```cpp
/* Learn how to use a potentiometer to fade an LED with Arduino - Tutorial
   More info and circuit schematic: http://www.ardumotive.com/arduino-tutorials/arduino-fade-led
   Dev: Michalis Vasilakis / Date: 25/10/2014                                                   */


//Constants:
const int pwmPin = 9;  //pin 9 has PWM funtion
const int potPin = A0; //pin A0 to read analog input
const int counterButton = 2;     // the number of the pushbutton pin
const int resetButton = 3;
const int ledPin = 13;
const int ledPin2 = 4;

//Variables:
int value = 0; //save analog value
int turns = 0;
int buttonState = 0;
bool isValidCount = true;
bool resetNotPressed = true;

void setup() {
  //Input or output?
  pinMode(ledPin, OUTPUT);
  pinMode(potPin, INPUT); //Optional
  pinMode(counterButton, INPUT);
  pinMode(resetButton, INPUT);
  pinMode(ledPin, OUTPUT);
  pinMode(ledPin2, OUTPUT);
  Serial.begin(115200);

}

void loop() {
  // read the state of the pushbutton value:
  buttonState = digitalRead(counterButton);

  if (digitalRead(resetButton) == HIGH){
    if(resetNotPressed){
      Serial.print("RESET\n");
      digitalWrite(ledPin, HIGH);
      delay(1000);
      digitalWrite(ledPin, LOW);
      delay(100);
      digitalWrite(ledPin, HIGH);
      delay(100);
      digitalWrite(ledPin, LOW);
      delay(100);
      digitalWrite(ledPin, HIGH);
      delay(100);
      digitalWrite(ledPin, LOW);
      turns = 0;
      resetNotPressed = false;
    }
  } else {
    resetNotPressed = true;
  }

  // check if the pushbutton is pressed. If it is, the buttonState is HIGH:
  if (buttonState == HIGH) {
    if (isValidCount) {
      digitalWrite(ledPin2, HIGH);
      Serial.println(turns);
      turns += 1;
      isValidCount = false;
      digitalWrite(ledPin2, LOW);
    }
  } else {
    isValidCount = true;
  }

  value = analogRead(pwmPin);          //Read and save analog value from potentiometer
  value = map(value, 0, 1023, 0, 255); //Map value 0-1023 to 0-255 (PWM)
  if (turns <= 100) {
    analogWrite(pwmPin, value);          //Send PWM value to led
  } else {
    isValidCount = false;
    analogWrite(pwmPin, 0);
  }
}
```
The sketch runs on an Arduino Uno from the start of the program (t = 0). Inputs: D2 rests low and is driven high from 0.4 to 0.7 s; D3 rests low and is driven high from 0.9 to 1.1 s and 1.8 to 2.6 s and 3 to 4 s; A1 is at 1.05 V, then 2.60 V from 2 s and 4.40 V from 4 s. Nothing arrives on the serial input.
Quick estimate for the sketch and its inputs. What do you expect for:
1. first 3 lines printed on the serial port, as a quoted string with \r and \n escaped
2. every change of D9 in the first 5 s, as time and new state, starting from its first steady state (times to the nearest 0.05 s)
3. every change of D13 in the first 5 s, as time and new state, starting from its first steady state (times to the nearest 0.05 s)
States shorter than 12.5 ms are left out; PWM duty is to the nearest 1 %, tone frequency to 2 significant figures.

"0\r\nRESET\nRESET\n"
0 s PWM 21 %; 2.3 s PWM 52 %; 4.4 s PWM 88 %
0 s low; 0.9 s high; 1.9 s low; 2 s high; 2.1 s low; 2.2 s high; 2.3 s low; 3 s high; 4 s low; 4.1 s high; 4.2 s low; 4.3 s high; 4.4 s low
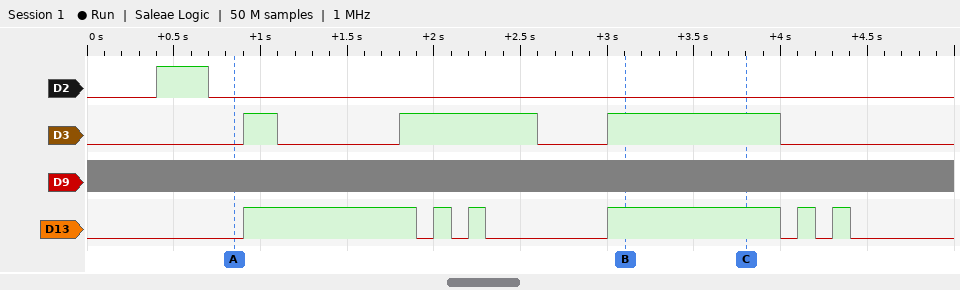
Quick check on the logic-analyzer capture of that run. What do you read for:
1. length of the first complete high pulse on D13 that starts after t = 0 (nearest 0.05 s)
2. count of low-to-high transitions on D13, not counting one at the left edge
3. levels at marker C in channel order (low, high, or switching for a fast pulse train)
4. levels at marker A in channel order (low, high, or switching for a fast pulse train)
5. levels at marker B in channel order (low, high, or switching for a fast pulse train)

1.00 s
6
D2 low, D3 high, D9 switching, D13 high
D2 low, D3 low, D9 switching, D13 low
D2 low, D3 high, D9 switching, D13 high
